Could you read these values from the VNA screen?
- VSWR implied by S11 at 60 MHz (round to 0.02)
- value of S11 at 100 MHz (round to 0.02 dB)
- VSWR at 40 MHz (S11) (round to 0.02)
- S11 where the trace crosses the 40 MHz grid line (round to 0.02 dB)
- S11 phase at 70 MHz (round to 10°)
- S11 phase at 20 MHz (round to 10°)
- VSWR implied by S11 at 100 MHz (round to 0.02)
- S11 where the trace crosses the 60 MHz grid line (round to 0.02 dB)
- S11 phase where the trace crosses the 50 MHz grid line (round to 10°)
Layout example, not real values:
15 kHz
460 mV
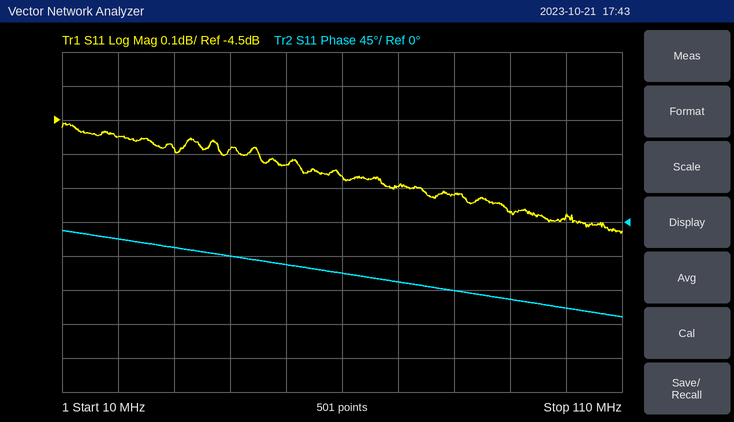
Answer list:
3.82
-4.78 dB
3.88
-4.58 dB
-80°
-20°
3.72
-4.66 dB
-60°
